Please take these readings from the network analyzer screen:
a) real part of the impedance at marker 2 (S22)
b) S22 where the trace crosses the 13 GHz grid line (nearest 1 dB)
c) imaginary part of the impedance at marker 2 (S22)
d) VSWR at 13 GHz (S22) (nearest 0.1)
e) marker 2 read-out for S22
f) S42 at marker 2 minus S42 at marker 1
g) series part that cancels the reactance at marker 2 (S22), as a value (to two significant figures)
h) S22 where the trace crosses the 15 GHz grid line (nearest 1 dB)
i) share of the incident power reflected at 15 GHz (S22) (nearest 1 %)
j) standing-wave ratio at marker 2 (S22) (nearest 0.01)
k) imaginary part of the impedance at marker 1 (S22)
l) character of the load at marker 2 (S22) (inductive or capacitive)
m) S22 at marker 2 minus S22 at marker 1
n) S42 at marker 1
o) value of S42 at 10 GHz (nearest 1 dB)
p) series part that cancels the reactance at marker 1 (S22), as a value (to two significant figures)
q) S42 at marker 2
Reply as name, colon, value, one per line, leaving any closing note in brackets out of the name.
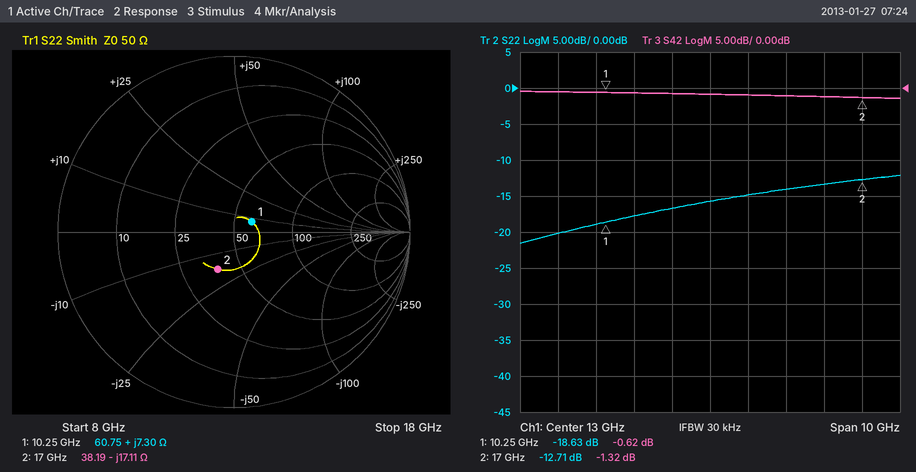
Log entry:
real part of the impedance at marker 2: 38.19 Ω
S22 where the trace crosses the 13 GHz grid line: -16 dB
imaginary part of the impedance at marker 2: -17.11 Ω
VSWR at 13 GHz (S22): 1.4
marker 2 read-out for S22: -12.71 dB
S42 at marker 2 minus S42 at marker 1: -0.70 dB
series part that cancels the reactance at marker 2 (S22), as a value: 160 pH
S22 where the trace crosses the 15 GHz grid line: -14 dB
share of the incident power reflected at 15 GHz (S22): 4 %
standing-wave ratio at marker 2 (S22): 1.60
imaginary part of the impedance at marker 1: +7.30 Ω
character of the load at marker 2 (S22): capacitive
S22 at marker 2 minus S22 at marker 1: 5.92 dB
S42 at marker 1: -0.62 dB
value of S42 at 10 GHz: -1 dB
series part that cancels the reactance at marker 1 (S22), as a value: 2.1 pF
S42 at marker 2: -1.32 dB
